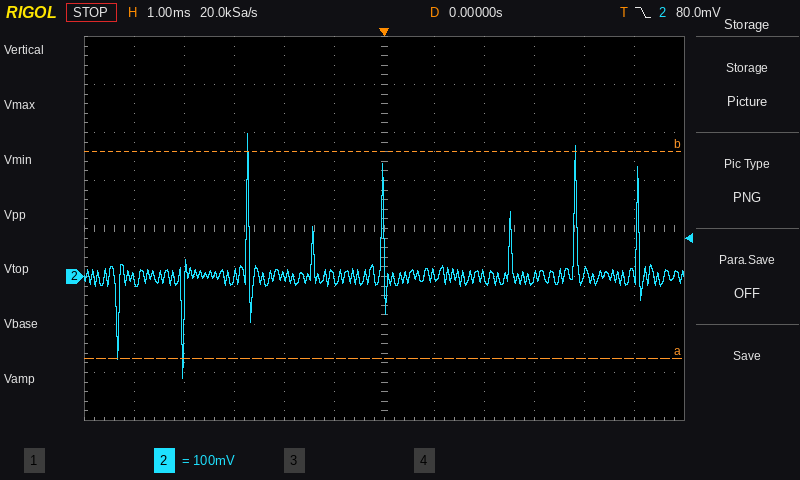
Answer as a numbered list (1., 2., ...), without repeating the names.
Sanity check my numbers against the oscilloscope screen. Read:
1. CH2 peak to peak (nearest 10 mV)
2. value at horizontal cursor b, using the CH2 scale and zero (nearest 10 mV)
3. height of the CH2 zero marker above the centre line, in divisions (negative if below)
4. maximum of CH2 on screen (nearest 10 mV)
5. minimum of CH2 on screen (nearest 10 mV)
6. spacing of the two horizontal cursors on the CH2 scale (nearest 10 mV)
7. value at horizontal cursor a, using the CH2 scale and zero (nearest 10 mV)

1. 510 mV
2. 260 mV
3. -1.0 div
4. 300 mV
5. -210 mV
6. 430 mV
7. -170 mV
